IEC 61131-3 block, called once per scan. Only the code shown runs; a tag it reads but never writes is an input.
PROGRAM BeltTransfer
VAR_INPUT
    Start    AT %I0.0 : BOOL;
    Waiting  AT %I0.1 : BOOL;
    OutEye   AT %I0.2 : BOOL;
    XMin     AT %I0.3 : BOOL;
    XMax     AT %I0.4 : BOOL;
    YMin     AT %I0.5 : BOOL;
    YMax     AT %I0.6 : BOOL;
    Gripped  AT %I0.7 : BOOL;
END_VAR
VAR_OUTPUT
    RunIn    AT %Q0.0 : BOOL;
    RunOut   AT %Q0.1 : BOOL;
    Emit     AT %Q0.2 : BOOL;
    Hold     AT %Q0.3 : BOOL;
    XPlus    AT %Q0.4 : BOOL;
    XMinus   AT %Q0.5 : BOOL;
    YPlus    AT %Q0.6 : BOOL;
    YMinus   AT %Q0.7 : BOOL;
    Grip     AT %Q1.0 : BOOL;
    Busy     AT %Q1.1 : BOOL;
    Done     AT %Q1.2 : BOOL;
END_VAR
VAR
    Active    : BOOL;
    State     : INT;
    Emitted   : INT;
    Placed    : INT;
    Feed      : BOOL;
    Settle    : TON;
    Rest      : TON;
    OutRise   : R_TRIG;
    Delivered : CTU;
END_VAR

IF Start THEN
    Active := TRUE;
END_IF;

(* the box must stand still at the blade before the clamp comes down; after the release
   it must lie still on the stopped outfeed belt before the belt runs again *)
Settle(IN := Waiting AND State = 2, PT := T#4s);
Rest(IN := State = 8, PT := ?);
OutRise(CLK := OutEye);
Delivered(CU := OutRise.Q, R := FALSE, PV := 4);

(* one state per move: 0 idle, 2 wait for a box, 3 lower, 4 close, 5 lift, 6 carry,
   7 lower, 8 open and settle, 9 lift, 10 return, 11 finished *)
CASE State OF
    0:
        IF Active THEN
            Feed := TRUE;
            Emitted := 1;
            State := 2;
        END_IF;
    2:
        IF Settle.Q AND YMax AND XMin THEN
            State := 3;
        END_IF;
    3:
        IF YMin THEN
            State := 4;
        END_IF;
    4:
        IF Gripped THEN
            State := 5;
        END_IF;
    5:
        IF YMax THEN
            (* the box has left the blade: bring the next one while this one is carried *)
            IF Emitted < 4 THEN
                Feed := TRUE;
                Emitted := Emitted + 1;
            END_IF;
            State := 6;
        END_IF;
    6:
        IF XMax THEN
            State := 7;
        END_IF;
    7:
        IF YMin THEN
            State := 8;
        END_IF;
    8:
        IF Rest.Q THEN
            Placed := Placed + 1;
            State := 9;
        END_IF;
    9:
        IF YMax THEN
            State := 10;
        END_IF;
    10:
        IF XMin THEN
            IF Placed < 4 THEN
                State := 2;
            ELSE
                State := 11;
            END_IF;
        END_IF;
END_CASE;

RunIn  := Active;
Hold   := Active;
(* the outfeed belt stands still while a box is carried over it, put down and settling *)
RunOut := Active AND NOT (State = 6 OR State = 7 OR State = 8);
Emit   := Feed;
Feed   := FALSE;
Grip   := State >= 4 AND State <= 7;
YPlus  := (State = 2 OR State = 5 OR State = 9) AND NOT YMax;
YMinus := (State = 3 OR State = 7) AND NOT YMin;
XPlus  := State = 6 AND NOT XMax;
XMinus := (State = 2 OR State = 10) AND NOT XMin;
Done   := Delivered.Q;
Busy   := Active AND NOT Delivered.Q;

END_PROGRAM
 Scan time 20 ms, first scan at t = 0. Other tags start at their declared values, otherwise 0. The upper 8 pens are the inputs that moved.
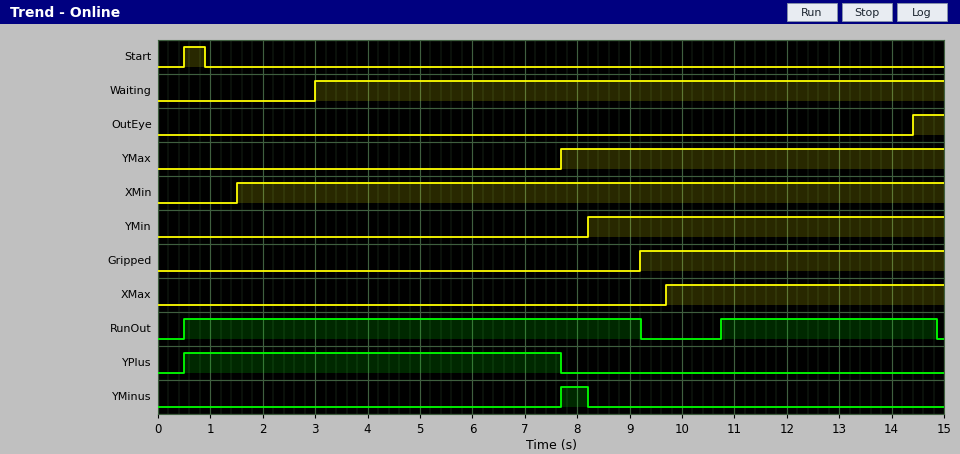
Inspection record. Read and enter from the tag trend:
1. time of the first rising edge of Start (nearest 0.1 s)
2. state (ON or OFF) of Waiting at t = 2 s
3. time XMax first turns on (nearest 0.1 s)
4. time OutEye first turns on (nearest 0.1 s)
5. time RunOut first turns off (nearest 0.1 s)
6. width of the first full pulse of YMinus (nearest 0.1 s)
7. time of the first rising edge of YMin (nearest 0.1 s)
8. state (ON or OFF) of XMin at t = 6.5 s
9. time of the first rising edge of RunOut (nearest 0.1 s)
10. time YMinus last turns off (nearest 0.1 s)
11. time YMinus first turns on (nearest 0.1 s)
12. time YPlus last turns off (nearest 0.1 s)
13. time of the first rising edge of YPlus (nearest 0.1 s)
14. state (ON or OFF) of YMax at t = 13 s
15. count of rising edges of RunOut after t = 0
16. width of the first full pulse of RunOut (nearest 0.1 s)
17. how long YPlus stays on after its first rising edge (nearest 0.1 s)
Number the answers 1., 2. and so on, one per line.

1. 0.5 s
2. OFF
3. 9.7 s
4. 14.4 s
5. 9.2 s
6. 0.5 s
7. 8.2 s
8. ON
9. 0.5 s
10. 8.2 s
11. 7.7 s
12. 7.7 s
13. 0.5 s
14. ON
15. 2
16. 8.7 s
17. 7.2 s
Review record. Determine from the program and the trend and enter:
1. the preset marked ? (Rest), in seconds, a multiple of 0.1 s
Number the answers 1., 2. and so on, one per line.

1. 1.0 s
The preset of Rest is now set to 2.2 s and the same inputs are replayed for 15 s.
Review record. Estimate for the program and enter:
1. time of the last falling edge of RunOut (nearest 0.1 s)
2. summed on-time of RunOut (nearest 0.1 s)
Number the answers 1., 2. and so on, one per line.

1. 9.2 s
2. 11.8 s
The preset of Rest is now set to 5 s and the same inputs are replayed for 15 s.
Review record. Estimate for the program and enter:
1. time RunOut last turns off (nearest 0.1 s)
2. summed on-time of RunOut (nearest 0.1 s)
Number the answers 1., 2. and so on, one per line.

1. 9.2 s
2. 9.0 s
